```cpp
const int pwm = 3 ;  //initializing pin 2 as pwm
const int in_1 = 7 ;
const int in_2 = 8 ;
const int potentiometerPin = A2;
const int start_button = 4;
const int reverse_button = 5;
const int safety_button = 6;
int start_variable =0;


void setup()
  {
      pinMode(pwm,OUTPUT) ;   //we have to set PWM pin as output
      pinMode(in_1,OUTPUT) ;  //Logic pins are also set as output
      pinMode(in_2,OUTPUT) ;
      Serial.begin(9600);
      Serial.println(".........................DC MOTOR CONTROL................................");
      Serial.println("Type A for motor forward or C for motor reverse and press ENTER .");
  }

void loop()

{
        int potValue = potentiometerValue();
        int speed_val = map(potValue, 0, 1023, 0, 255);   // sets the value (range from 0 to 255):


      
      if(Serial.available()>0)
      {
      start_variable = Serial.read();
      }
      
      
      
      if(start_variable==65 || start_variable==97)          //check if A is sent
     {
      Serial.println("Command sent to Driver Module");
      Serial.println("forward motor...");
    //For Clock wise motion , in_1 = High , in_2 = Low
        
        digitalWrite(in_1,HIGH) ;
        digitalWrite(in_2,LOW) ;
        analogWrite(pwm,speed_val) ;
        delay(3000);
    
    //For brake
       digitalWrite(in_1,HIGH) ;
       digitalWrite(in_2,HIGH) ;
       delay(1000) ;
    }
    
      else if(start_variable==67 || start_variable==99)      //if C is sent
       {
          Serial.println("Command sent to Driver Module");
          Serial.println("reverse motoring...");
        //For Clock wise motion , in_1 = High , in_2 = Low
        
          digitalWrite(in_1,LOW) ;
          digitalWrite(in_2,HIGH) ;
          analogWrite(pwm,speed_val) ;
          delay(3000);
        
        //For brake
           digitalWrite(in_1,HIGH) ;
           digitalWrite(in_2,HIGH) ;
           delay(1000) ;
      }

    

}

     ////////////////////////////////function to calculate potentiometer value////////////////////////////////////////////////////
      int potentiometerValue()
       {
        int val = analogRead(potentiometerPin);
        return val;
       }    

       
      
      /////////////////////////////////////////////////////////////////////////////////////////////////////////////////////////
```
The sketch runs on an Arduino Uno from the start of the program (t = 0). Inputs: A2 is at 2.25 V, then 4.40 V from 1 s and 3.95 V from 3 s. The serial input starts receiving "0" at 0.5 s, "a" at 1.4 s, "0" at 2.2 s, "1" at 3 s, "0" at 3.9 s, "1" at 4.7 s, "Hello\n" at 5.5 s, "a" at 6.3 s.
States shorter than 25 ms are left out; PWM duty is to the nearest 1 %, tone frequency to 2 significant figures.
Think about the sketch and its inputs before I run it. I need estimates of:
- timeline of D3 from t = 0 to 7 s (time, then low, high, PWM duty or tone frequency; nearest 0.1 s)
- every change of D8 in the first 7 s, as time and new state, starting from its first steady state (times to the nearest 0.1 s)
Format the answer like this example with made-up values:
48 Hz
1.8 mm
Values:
0 s low; 1.4 s PWM 88 %; 6.3 s PWM 79 %
0 s low; 4.4 s high; 6.3 s low
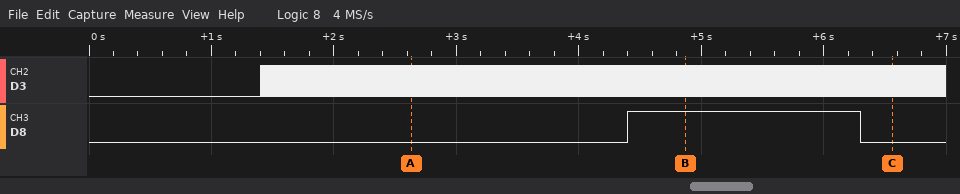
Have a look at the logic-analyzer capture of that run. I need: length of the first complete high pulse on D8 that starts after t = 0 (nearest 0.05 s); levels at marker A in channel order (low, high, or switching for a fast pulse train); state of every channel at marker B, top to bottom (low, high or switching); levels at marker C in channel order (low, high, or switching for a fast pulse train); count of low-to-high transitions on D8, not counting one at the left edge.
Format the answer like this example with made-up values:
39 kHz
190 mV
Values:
1.90 s
D3 switching, D8 low
D3 switching, D8 high
D3 switching, D8 low
1
